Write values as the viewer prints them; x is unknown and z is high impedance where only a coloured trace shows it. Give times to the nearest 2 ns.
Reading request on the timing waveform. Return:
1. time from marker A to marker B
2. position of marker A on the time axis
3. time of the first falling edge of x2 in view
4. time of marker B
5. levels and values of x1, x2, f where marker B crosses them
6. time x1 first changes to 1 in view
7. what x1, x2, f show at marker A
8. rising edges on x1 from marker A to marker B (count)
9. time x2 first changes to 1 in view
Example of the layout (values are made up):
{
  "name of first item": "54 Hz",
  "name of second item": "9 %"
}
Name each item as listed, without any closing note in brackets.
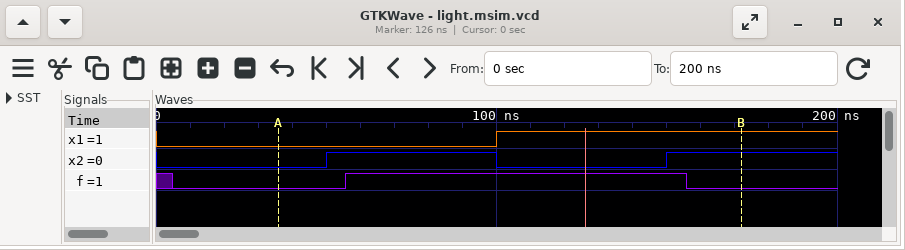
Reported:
{
  "time from marker A to marker B": "136 ns",
  "position of marker A on the time axis": "36 ns",
  "time of the first falling edge of x2 in view": "100 ns",
  "time of marker B": "172 ns",
  "levels and values of x1, x2, f where marker B crosses them": "x1=1, x2=1, f=0",
  "time x1 first changes to 1 in view": "100 ns",
  "what x1, x2, f show at marker A": "x1=0, x2=0, f=0",
  "rising edges on x1 from marker A to marker B": "1",
  "time x2 first changes to 1 in view": "50 ns"
}
